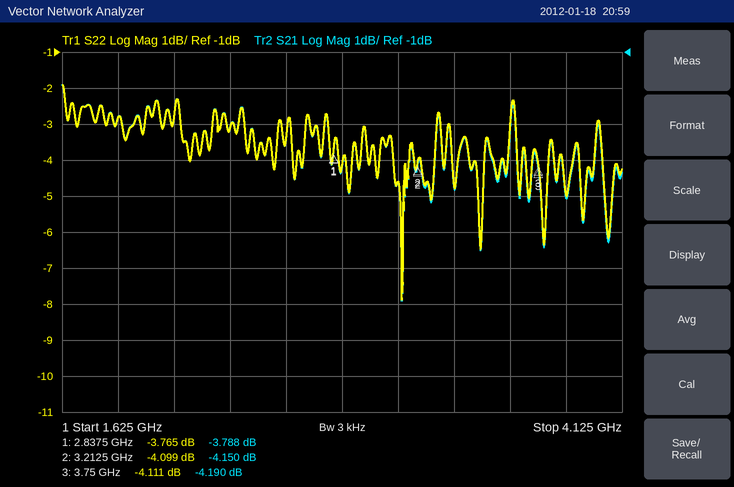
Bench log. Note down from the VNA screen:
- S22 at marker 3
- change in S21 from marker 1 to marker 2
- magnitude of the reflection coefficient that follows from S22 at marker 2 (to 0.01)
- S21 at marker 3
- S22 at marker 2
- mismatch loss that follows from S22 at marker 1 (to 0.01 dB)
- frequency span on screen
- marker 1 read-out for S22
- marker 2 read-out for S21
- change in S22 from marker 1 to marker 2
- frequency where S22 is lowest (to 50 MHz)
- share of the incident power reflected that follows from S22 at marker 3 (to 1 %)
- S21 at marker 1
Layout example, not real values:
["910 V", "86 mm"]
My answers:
["-4.111 dB", "-0.362 dB", "0.62", "-4.190 dB", "-4.099 dB", "2.37 dB", "2.5 GHz", "-3.765 dB", "-4.150 dB", "-0.334 dB", "3.15 GHz", "39 %", "-3.788 dB"]
